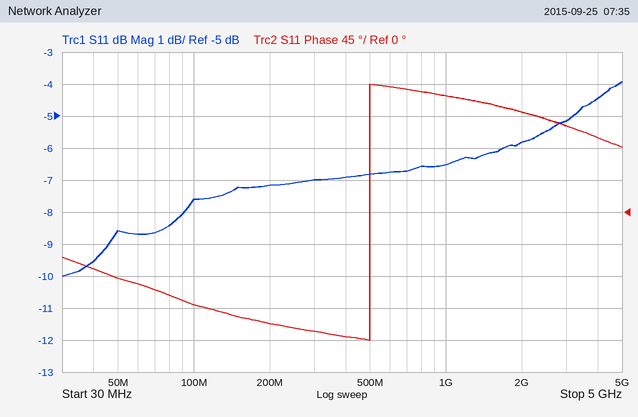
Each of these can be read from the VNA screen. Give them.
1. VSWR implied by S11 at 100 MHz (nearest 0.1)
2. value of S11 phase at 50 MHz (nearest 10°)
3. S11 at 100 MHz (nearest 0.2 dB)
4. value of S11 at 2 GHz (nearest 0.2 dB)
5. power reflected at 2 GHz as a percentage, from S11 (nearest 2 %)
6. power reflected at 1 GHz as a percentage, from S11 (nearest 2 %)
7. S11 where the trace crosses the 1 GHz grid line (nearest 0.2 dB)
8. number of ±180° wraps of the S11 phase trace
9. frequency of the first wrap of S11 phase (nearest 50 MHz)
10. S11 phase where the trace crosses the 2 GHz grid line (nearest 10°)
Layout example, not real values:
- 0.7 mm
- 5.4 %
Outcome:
- 2.4
- -90°
- -7.6 dB
- -5.8 dB
- 26 %
- 22 %
- -6.6 dB
- 1
- 500 MHz
- 140°
